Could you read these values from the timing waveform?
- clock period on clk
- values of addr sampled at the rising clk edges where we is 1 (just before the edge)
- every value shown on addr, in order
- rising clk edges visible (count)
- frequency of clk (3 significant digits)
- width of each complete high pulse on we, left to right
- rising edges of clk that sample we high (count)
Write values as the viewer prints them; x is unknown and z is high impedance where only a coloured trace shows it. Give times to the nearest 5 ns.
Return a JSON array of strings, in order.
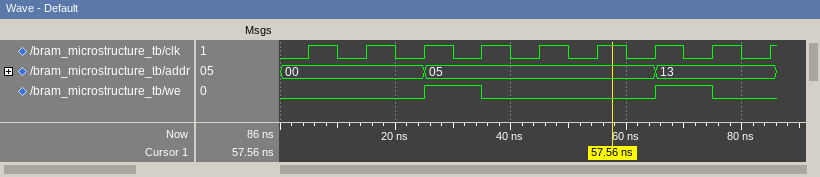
["10 ns", "05, 13", "00, 05, 13", "9", "100 MHz", "10 ns, 10 ns", "2"]
